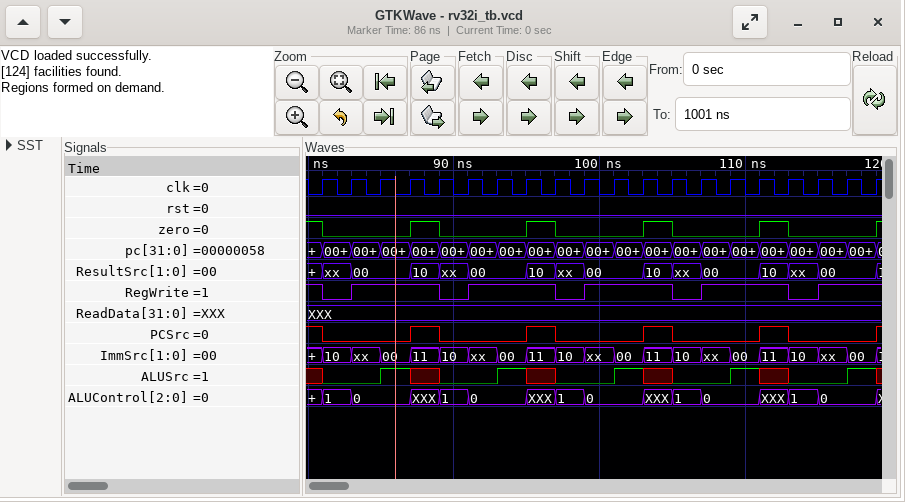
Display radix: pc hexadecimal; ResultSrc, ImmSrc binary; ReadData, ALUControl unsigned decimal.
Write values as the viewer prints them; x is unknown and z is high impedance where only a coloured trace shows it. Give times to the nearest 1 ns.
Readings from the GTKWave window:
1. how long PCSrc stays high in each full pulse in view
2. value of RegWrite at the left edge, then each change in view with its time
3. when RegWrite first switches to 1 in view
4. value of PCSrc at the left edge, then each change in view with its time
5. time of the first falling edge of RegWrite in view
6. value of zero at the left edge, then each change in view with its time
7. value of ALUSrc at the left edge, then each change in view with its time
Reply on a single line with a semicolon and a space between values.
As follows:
2 ns, 2 ns, 2 ns, 2 ns; 1, 0 at 81 ns, 1 at 83 ns, 0 at 89 ns, 1 at 91 ns, 0 at 97 ns, 1 at 99 ns, 0 at 105 ns, 1 at 107 ns, 0 at 113 ns, 1 at 115 ns; 83 ns; 1, 0 at 81 ns, 1 at 87 ns, 0 at 89 ns, 1 at 95 ns, 0 at 97 ns, 1 at 103 ns, 0 at 105 ns, 1 at 111 ns, 0 at 113 ns, 1 at 119 ns; 81 ns; 1, 0 at 81 ns, 1 at 87 ns, 0 at 89 ns, 1 at 95 ns, 0 at 97 ns, 1 at 103 ns, 0 at 105 ns, 1 at 111 ns, 0 at 113 ns, 1 at 119 ns; x, 0 at 81 ns, 1 at 85 ns, x at 87 ns, 0 at 89 ns, 1 at 93 ns, x at 95 ns, 0 at 97 ns, 1 at 101 ns, x at 103 ns, 0 at 105 ns, 1 at 109 ns, x at 111 ns, 0 at 113 ns, 1 at 117 ns, x at 119 ns
